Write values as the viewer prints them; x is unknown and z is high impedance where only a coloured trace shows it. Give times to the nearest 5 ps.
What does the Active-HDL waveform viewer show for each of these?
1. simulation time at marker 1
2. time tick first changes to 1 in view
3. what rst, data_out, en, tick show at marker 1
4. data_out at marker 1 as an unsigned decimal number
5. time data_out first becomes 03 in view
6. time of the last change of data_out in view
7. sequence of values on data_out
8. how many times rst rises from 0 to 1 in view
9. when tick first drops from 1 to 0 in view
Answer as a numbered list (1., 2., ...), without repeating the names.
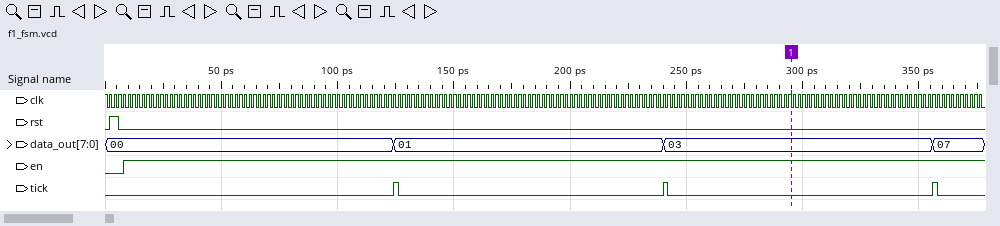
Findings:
1. 295 ps
2. 125 ps
3. rst=0, data_out=03, en=1, tick=0
4. 3
5. 240 ps
6. 355 ps
7. 00, 01, 03, 07
8. 1
9. 125 ps
